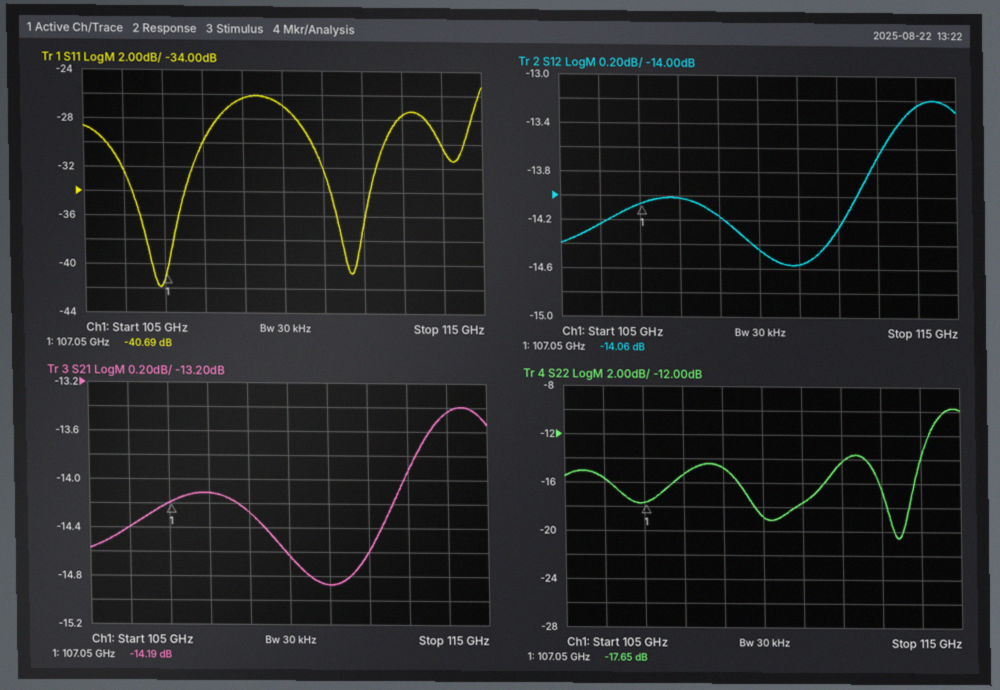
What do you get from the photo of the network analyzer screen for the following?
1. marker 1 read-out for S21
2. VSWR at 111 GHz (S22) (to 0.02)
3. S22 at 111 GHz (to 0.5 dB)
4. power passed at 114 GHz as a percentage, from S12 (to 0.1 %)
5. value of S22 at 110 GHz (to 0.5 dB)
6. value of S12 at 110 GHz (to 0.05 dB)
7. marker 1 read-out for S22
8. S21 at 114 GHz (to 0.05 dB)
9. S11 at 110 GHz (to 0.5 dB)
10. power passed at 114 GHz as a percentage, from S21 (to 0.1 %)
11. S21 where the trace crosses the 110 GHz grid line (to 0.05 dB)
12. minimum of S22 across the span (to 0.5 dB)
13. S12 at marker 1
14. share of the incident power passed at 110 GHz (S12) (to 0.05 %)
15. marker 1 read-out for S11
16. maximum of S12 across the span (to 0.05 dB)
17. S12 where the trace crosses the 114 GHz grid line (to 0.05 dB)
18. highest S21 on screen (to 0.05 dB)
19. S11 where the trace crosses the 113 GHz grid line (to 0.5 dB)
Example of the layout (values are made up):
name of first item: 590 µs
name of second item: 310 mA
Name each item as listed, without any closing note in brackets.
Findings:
marker 1 read-out for S21: -14.19 dB
VSWR at 111 GHz (S22): 1.30
S22 at 111 GHz: -17.5 dB
power passed at 114 GHz as a percentage, from S12: 4.7 %
value of S22 at 110 GHz: -19.0 dB
value of S12 at 110 GHz: -14.45 dB
marker 1 read-out for S22: -17.65 dB
S21 at 114 GHz: -13.45 dB
S11 at 110 GHz: -27.0 dB
power passed at 114 GHz as a percentage, from S21: 4.5 %
S21 where the trace crosses the 110 GHz grid line: -14.65 dB
minimum of S22 across the span: -20.5 dB
S12 at marker 1: -14.06 dB
share of the incident power passed at 110 GHz (S12): 3.60 %
marker 1 read-out for S11: -40.69 dB
maximum of S12 across the span: -13.20 dB
S12 where the trace crosses the 114 GHz grid line: -13.25 dB
highest S21 on screen: -13.40 dB
S11 where the trace crosses the 113 GHz grid line: -27.5 dB
